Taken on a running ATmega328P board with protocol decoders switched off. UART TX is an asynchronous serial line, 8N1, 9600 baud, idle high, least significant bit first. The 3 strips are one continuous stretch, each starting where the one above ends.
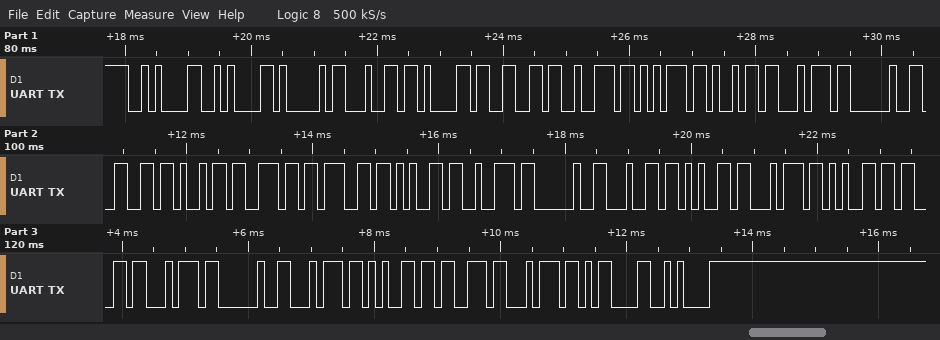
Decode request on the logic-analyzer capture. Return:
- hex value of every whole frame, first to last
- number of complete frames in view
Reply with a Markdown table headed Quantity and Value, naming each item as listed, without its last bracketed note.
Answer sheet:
| Quantity | Value |
|---|---|
| hex value of every whole frame, first to last | 0A 0A 41 64 61 66 72 75 69 74 20 66 69 6E 67 65 72 20 64 65 74 65 63 74 20 74 65 73 74 0D 0A |
| number of complete frames in view | 31 |
